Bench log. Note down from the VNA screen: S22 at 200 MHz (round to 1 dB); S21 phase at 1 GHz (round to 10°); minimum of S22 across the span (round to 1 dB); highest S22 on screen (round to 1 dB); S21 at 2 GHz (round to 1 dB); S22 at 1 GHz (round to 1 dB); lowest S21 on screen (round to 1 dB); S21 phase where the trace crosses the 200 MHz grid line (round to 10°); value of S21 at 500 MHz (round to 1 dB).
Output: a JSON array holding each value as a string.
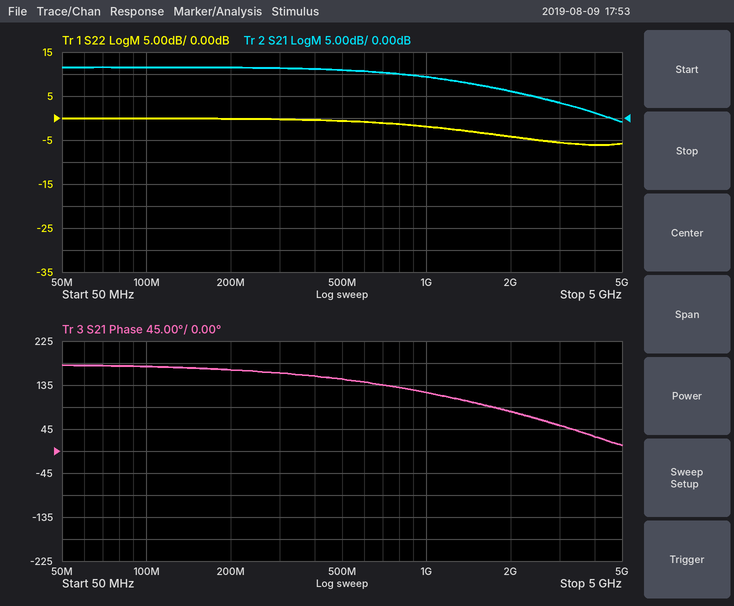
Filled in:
["0 dB", "120°", "-6 dB", "0 dB", "6 dB", "-2 dB", "-1 dB", "170°", "11 dB"]
